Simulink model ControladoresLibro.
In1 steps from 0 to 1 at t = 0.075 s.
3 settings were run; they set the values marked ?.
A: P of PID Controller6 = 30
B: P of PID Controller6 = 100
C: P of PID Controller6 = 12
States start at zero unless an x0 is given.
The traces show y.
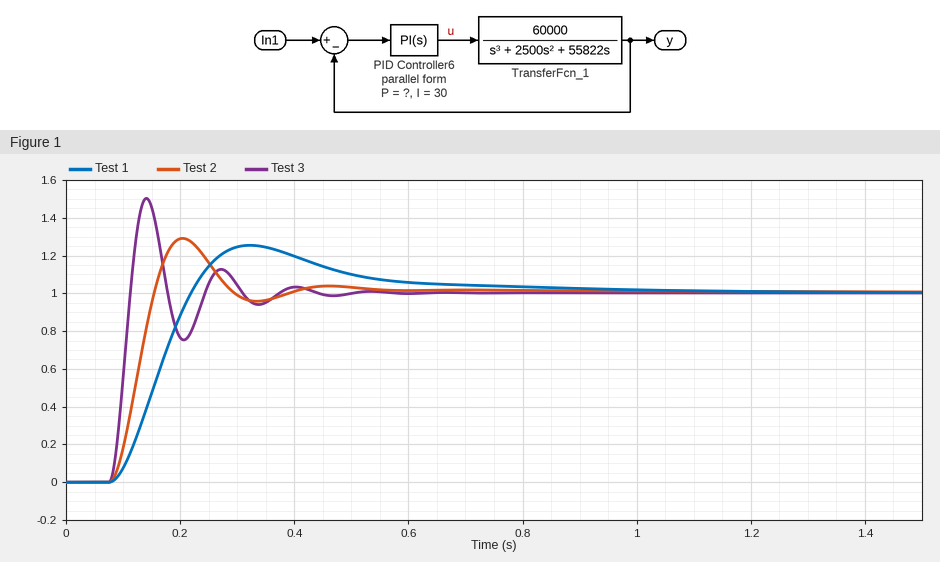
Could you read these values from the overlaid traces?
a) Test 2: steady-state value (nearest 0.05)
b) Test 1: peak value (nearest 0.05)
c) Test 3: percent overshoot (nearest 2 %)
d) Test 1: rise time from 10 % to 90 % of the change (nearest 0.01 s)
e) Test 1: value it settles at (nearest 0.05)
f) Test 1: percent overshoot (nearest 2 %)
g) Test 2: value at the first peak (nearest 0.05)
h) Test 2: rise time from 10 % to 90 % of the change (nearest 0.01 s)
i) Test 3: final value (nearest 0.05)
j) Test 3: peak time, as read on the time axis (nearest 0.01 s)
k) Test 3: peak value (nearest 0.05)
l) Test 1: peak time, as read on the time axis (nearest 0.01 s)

1.00
1.25
50 %
0.10 s
1.00
26 %
1.30
0.05 s
1.00
0.14 s
1.50
0.32 s
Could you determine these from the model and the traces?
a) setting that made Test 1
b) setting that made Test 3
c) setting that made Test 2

C
B
A
